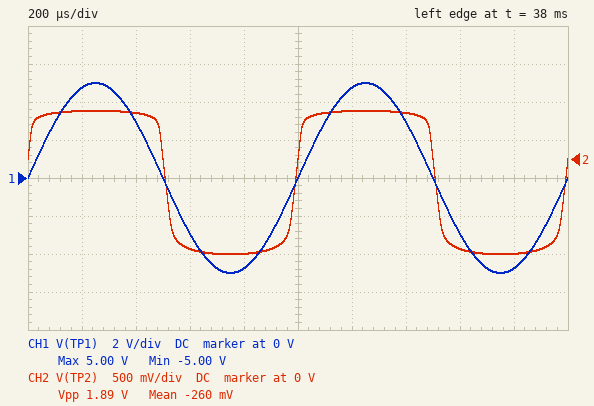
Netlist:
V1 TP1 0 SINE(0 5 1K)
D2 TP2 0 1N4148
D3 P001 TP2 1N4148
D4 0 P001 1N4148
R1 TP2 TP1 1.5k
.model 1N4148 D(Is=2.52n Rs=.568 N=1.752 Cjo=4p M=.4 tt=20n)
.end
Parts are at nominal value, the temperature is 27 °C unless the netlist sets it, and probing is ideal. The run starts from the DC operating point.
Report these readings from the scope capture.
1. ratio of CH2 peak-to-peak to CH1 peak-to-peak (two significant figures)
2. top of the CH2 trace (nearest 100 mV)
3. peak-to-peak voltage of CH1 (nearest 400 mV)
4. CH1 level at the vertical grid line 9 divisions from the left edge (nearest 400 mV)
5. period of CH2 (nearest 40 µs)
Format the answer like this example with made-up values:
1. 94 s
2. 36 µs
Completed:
1. 0.19
2. 600 mV
3. 10.0 V
4. -4.8 V
5. 1.00 ms
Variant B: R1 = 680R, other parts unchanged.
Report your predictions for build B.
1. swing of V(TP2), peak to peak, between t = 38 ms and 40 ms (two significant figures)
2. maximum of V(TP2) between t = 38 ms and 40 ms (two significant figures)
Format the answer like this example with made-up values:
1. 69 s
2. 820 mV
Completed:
1. 2.0 V
2. 670 mV
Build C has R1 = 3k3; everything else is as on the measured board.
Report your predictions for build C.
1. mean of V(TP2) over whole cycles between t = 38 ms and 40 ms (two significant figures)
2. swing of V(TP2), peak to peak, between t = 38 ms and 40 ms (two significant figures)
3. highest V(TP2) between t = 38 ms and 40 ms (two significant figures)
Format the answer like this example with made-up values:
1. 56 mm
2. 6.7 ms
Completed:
1. -250 mV
2. 1.8 V
3. 600 mV
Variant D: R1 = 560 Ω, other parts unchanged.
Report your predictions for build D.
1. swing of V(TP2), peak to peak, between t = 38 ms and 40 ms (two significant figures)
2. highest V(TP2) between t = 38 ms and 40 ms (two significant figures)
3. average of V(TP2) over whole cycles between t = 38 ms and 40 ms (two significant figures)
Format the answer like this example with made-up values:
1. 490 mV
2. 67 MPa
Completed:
1. 2.0 V
2. 680 mV
3. -280 mV
